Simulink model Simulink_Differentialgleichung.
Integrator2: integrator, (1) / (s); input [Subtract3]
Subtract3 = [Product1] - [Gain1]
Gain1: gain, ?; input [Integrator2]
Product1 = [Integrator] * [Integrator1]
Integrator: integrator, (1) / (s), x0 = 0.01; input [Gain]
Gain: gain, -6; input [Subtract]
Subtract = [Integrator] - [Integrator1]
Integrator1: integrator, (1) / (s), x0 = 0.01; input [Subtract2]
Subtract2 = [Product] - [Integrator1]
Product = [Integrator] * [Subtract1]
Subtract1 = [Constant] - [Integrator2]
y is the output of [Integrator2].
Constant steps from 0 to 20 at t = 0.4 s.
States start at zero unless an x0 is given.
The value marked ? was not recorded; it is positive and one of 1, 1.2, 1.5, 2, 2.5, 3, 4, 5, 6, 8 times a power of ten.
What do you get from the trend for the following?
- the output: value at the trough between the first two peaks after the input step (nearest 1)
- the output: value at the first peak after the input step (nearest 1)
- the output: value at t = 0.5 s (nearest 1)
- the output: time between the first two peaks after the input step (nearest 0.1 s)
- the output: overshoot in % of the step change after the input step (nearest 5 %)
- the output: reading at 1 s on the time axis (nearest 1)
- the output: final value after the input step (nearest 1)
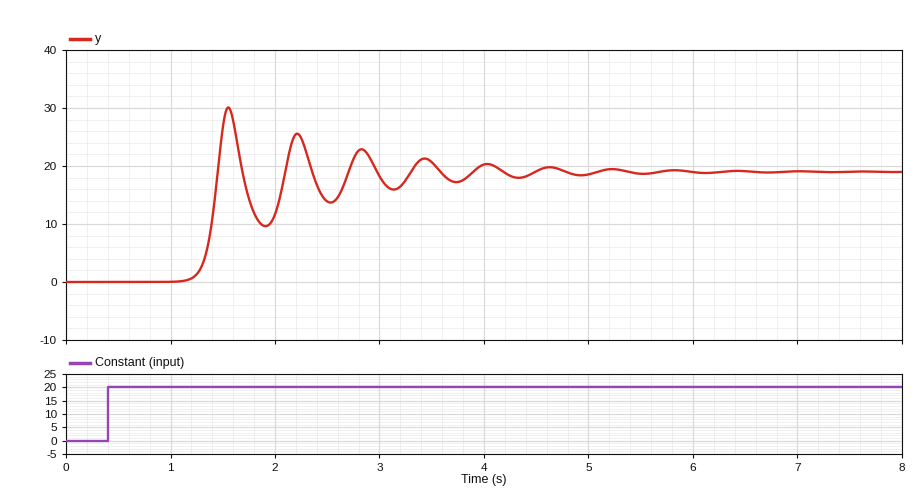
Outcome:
10
30
0
0.7 s
60 %
0
19
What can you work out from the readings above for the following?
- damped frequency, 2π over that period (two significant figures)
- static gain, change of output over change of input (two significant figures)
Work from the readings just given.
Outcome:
9.0 rad/s
0.95
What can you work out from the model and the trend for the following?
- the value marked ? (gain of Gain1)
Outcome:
5
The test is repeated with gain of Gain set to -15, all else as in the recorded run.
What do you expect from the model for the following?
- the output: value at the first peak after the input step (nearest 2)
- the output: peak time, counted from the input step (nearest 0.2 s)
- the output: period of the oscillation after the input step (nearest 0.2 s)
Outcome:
32
0.8 s
0.6 s
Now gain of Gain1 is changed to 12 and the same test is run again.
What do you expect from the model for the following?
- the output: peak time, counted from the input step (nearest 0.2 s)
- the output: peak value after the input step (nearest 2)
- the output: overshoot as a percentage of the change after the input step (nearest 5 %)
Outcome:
1.2 s
26
40 %
